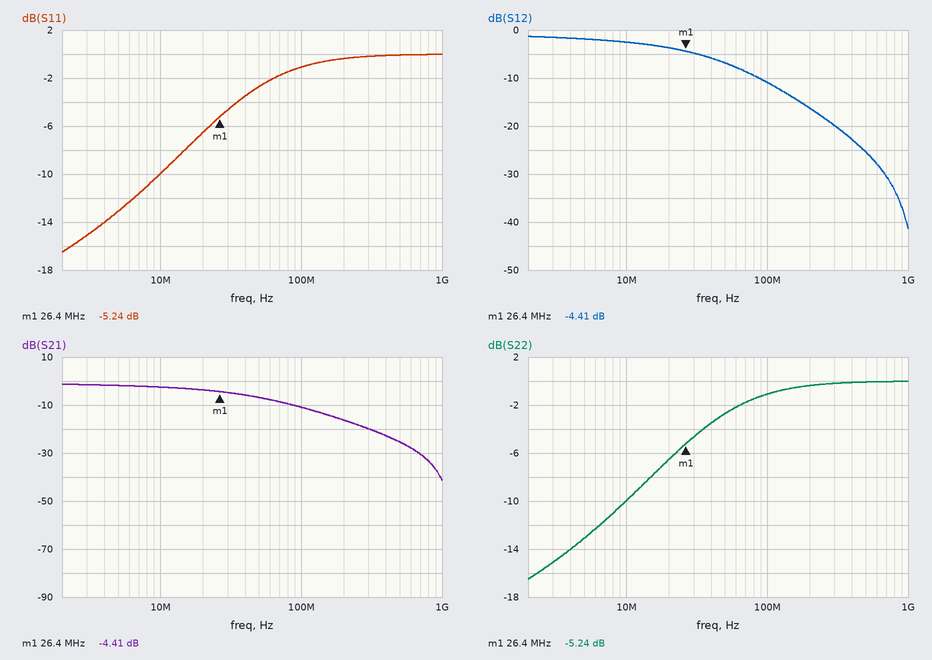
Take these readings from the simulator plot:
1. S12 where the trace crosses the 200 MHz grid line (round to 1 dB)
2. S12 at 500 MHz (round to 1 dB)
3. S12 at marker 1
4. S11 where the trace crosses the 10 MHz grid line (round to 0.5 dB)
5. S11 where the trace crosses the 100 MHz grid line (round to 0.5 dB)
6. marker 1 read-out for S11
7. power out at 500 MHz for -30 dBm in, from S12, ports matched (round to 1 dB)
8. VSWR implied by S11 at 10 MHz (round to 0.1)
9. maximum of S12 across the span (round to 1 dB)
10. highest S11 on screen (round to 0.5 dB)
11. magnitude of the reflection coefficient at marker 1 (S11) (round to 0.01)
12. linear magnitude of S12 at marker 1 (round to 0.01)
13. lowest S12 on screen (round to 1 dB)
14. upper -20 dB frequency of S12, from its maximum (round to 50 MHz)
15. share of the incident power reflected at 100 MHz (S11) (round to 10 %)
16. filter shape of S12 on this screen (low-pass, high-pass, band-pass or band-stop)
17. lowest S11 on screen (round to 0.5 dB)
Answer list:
-16 dB
-25 dB
-4.41 dB
-10.0 dB
-1.0 dB
-5.24 dB
-55 dBm
1.9
-1 dB
0.0 dB
0.55
0.60
-41 dB
350 MHz
80 %
low-pass
-16.5 dB
